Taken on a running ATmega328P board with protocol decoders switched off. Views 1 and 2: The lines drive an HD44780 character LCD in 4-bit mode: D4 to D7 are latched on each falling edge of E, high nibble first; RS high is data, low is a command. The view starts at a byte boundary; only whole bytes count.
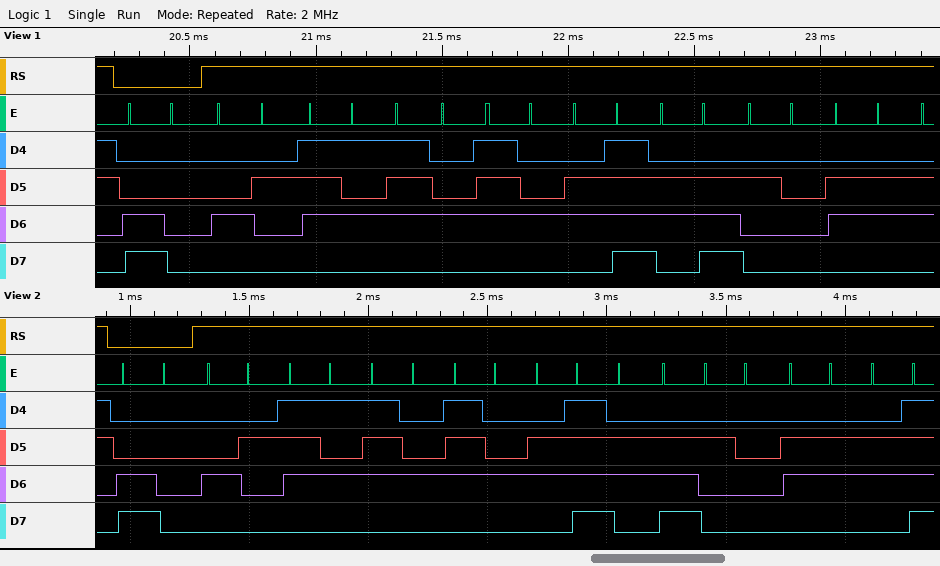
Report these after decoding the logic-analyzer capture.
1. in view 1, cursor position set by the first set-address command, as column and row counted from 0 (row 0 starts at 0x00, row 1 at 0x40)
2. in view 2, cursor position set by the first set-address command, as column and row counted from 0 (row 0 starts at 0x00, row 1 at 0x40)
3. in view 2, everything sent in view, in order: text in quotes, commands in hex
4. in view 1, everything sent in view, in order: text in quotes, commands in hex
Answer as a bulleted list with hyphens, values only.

- column 0, row 1
- column 0, row 1
- 0xC0 "Button fo"
- 0xC0 "Button f"
